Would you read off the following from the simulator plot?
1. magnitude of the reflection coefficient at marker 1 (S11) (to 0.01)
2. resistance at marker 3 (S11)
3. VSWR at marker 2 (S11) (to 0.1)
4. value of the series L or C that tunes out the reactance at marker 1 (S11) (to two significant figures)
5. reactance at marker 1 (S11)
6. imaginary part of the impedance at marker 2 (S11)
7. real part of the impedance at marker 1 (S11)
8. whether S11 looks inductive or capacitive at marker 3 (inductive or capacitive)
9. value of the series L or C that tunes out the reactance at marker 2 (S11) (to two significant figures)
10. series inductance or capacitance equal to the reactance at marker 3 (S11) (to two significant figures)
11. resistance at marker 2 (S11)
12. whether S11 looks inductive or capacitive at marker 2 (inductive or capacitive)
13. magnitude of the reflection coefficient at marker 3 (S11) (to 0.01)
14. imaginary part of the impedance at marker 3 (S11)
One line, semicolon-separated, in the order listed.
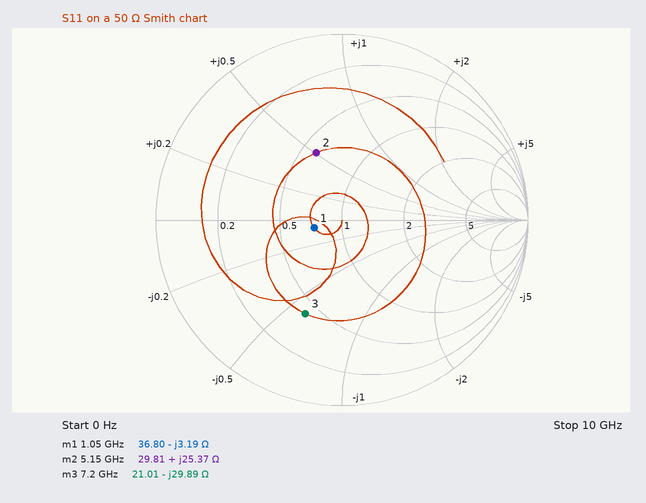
0.16; 21.01 Ω; 2.3; 480 pH; -3.19 Ω; +25.37 Ω; 36.80 Ω; capacitive; 1.2 pF; 740 fF; 29.81 Ω; inductive; 0.54; -29.89 Ω
